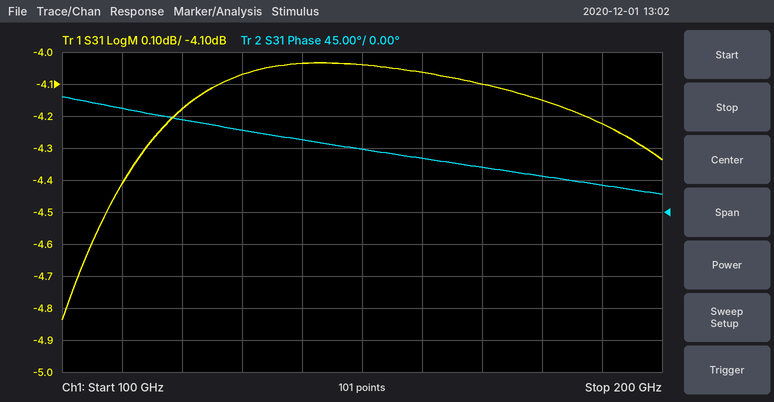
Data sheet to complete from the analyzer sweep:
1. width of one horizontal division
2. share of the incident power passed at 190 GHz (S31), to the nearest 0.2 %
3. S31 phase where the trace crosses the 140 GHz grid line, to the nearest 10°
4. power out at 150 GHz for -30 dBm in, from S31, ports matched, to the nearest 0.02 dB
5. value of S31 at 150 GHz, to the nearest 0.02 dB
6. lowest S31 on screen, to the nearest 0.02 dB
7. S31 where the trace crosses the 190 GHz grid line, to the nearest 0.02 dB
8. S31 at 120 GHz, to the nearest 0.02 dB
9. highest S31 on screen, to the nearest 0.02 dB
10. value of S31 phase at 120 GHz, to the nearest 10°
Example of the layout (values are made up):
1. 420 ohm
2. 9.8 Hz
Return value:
1. 10 GHz
2. 37.8 %
3. 100°
4. -34.04 dBm
5. -4.04 dB
6. -4.84 dB
7. -4.22 dB
8. -4.18 dB
9. -4.04 dB
10. 130°
